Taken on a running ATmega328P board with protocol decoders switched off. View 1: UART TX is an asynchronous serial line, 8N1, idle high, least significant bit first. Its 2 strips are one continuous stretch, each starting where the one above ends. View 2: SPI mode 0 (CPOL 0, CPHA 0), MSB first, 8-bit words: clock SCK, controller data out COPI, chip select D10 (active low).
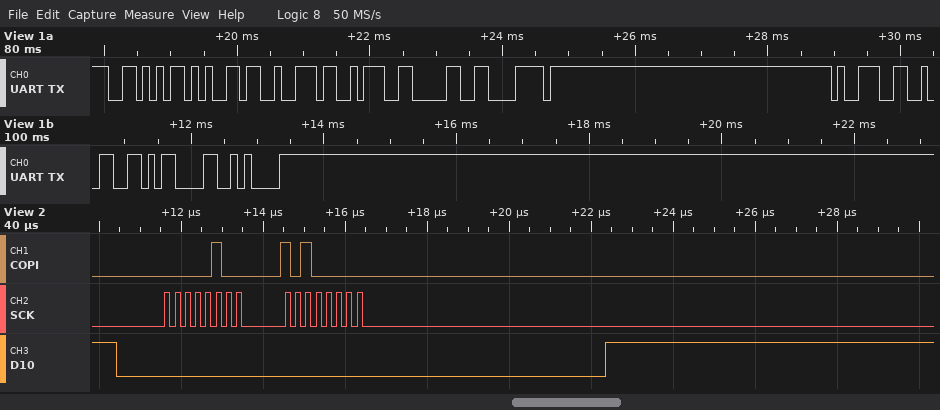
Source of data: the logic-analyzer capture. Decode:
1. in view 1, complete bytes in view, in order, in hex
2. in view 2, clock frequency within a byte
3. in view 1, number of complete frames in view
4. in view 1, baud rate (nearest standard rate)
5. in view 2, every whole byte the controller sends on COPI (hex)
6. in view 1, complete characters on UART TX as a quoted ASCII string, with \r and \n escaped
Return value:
56 65 72 3A 30 78 39 32 0D 0A
4 MHz
10
9600 baud
04 A0
"Ver:0x92\r\n"
